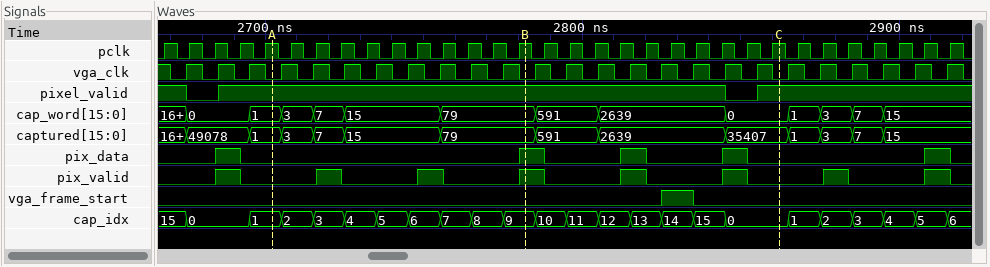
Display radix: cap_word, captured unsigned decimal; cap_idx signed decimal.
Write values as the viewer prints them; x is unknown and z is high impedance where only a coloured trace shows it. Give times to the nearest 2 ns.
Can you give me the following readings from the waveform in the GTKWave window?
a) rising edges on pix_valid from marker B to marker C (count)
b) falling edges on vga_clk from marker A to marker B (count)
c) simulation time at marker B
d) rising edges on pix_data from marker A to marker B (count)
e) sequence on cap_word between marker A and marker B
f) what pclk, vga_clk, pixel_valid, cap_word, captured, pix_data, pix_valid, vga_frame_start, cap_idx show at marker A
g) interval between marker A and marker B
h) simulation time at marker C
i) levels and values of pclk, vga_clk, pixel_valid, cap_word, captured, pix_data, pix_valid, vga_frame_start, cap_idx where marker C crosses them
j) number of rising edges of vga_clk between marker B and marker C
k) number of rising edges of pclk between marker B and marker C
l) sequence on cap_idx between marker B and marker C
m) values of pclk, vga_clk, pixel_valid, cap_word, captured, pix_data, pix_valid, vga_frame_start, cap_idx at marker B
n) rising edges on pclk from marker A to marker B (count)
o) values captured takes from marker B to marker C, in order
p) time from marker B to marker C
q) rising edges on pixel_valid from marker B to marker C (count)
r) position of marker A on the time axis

2
8
2782 ns
1
1, 3, 7, 15, 79
pclk=1, vga_clk=0, pixel_valid=1, cap_word=1, captured=1, pix_data=0, pix_valid=0, vga_frame_start=0, cap_idx=1
80 ns
2862 ns
pclk=1, vga_clk=0, pixel_valid=1, cap_word=0, captured=35407, pix_data=0, pix_valid=0, vga_frame_start=0, cap_idx=0
8
10
9, 10, 11, 12, 13, 14, 15, 0
pclk=1, vga_clk=0, pixel_valid=1, cap_word=79, captured=79, pix_data=1, pix_valid=1, vga_frame_start=0, cap_idx=9
10
79, 591, 2639, 35407
80 ns
1
2702 ns
